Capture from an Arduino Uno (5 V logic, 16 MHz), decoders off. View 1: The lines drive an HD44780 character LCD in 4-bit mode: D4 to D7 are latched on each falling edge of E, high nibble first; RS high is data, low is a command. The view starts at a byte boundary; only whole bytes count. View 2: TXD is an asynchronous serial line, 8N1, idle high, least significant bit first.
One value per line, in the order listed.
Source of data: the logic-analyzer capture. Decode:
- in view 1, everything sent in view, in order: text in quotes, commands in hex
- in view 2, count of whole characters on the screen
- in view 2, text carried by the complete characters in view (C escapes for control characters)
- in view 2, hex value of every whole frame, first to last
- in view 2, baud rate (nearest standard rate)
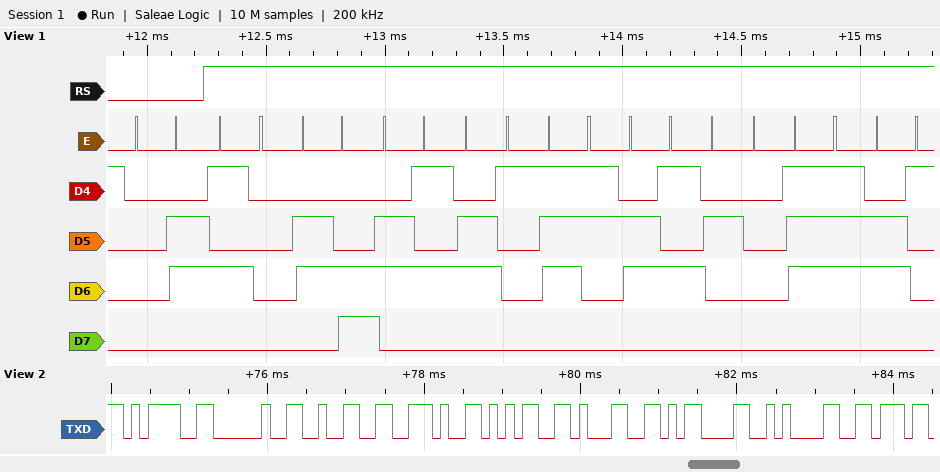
0x06 "Please wa"
9
"= 2.51\r\nv"
3D 20 32 2E 35 31 0D 0A 76
9600 baud
